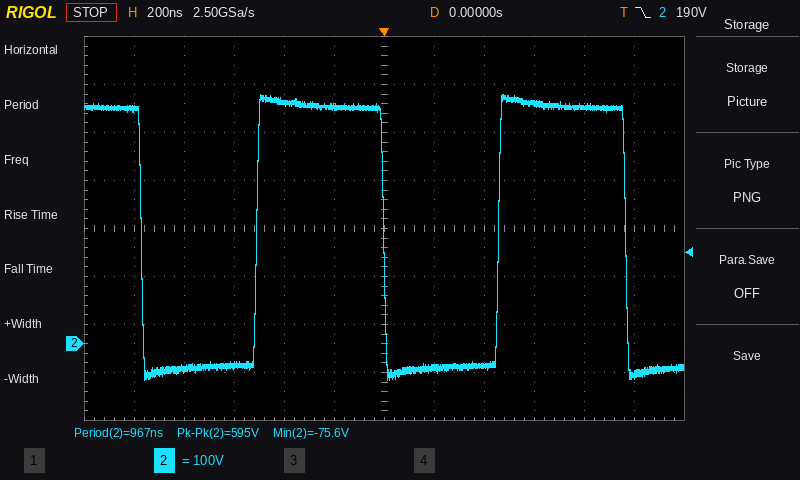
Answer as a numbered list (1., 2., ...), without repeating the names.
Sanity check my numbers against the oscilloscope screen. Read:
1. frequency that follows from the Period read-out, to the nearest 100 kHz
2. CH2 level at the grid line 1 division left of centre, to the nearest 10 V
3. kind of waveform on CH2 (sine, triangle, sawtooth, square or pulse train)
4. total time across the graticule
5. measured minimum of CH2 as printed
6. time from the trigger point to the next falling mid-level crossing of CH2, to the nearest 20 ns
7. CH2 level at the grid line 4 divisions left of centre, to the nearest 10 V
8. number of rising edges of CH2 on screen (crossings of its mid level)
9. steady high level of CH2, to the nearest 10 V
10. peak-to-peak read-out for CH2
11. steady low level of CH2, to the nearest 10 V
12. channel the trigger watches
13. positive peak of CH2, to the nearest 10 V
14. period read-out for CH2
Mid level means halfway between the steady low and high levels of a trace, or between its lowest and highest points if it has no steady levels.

1. 1.0 MHz
2. 490 V
3. square
4. 2.4 µs
5. -75.6 V
6. 960 ns
7. -50 V
8. 2
9. 490 V
10. 595 V
11. -50 V
12. CH2
13. 520 V
14. 967 ns
